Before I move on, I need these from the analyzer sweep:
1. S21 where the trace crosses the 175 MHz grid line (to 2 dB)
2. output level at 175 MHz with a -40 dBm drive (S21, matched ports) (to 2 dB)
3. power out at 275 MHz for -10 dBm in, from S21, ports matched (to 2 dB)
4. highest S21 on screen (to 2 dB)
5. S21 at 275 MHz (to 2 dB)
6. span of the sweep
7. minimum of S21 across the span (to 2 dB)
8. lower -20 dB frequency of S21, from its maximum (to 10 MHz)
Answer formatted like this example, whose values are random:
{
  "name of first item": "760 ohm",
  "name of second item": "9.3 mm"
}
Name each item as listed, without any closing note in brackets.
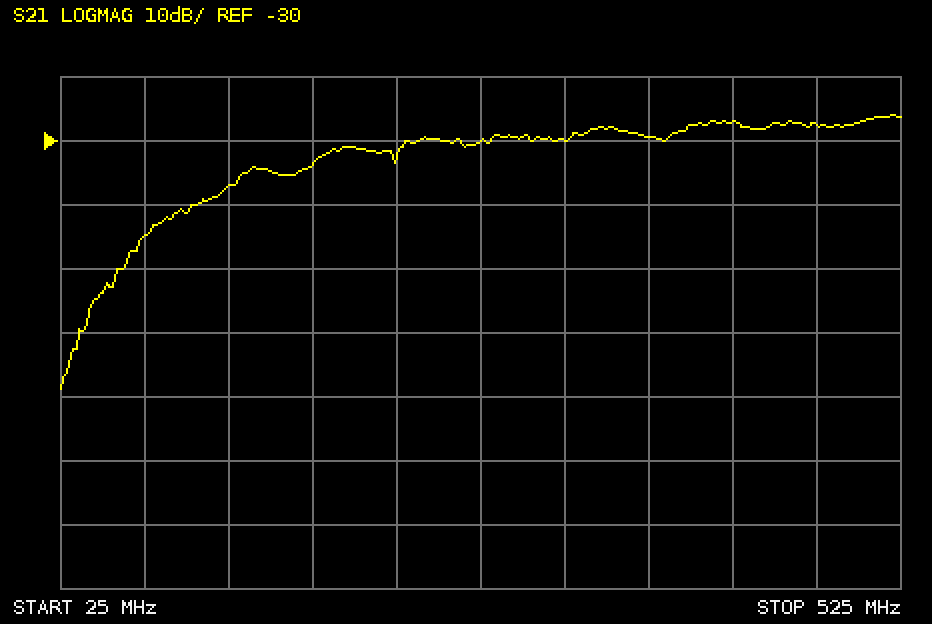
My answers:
{
  "S21 where the trace crosses the 175 MHz grid line": "-34 dB",
  "output level at 175 MHz with a -40 dBm drive (S21, matched ports)": "-74 dBm",
  "power out at 275 MHz for -10 dBm in, from S21, ports matched": "-40 dBm",
  "highest S21 on screen": "-26 dB",
  "S21 at 275 MHz": "-30 dB",
  "span of the sweep": "500 MHz",
  "minimum of S21 across the span": "-68 dB",
  "lower -20 dB frequency of S21, from its maximum": "70 MHz"
}
